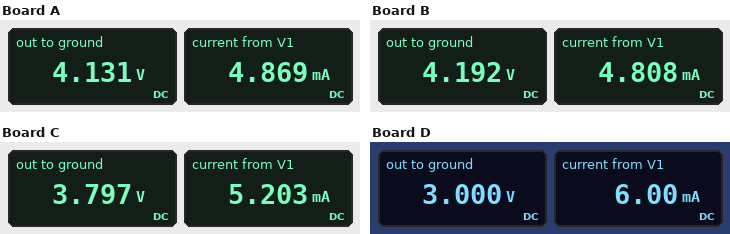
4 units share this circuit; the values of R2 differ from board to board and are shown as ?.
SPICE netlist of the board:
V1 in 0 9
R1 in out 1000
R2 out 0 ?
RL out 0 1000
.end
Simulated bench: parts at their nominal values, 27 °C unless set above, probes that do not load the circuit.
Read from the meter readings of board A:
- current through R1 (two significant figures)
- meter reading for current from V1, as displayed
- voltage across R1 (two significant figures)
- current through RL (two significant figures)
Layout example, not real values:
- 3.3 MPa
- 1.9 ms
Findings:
- 4.9 mA
- 4.869 mA
- 4.9 V
- 4.1 mA
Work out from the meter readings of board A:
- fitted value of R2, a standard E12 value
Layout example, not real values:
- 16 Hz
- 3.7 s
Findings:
- 5.6 kΩ
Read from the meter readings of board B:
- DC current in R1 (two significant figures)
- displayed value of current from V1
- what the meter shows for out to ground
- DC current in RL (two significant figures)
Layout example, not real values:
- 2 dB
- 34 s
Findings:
- 4.8 mA
- 4.808 mA
- 4.192 V
- 4.2 mA
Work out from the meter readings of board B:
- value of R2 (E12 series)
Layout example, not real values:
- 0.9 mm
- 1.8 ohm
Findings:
- 6.8 kΩ
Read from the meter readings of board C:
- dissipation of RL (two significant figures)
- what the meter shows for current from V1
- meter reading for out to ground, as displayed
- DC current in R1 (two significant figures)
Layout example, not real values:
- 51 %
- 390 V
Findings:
- 14 mW
- 5.203 mA
- 3.797 V
- 5.2 mA
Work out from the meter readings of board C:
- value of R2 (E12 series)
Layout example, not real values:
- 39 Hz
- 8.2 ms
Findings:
- 2.7 kΩ
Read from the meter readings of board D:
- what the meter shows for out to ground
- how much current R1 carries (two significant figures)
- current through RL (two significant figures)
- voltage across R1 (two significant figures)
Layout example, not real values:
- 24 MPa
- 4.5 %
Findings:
- 3.000 V
- 6.0 mA
- 3.0 mA
- 6.0 V
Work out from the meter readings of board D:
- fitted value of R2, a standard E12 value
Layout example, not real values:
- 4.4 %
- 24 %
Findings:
- 1 kΩ
